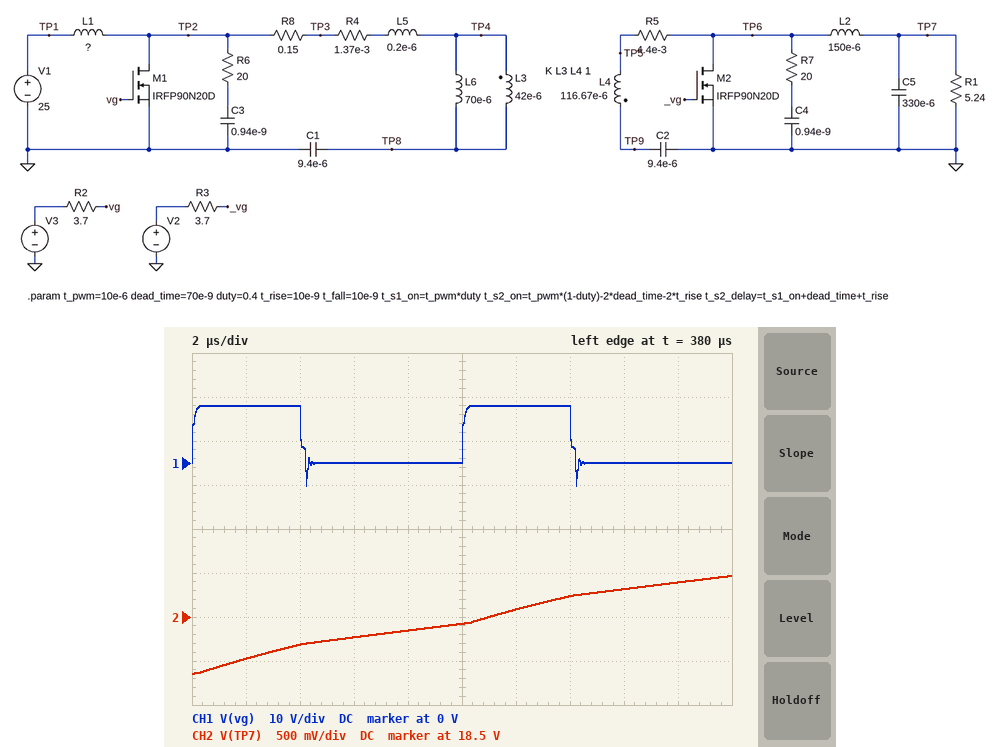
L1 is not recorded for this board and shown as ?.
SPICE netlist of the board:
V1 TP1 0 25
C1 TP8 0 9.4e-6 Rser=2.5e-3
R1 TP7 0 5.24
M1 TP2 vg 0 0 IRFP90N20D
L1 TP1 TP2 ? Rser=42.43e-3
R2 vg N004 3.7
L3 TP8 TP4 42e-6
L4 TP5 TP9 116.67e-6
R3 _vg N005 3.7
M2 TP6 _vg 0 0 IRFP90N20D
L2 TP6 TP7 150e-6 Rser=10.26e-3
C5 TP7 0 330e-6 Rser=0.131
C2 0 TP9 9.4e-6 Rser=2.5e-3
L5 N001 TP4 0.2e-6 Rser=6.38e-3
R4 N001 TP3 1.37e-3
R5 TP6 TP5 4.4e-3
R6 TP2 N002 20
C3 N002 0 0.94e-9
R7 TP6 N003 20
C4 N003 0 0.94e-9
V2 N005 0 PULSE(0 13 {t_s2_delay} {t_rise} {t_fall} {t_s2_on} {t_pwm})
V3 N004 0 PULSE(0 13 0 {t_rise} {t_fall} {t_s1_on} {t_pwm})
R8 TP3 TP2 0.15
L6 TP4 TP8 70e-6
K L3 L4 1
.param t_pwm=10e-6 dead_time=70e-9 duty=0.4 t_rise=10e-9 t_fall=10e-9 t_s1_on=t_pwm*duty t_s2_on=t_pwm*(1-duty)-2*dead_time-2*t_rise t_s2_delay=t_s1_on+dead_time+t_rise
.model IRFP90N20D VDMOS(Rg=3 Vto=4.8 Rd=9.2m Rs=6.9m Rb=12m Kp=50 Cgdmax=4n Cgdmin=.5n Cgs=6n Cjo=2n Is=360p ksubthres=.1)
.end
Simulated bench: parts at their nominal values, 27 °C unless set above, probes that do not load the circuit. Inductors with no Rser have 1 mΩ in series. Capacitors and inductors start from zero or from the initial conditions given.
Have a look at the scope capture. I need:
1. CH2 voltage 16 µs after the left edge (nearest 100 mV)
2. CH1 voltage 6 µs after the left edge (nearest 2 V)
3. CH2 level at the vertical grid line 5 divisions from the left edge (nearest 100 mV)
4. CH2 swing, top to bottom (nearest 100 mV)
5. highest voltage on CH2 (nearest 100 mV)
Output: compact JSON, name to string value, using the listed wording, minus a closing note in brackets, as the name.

{"CH2 voltage 16 µs after the left edge": "18.8 V", "CH1 voltage 6 µs after the left edge": "0 V", "CH2 level at the vertical grid line 5 divisions from the left edge": "18.4 V", "CH2 swing, top to bottom": "1.1 V", "highest voltage on CH2": "19.0 V"}
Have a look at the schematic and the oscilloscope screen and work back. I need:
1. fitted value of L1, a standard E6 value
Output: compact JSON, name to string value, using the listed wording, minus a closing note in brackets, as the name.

{"fitted value of L1, a standard E6 value": "47 µH"}
